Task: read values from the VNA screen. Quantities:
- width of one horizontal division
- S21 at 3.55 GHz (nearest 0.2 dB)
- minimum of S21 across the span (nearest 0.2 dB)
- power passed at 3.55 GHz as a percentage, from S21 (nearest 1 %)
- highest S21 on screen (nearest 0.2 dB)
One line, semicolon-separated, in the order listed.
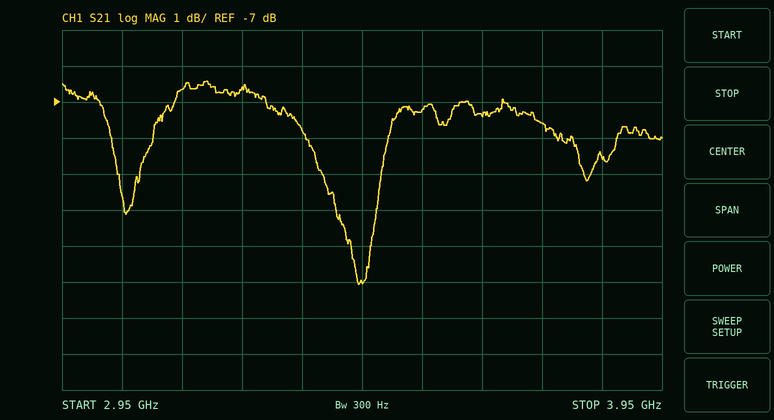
100 MHz; -7.2 dB; -12.0 dB; 19 %; -6.4 dB
